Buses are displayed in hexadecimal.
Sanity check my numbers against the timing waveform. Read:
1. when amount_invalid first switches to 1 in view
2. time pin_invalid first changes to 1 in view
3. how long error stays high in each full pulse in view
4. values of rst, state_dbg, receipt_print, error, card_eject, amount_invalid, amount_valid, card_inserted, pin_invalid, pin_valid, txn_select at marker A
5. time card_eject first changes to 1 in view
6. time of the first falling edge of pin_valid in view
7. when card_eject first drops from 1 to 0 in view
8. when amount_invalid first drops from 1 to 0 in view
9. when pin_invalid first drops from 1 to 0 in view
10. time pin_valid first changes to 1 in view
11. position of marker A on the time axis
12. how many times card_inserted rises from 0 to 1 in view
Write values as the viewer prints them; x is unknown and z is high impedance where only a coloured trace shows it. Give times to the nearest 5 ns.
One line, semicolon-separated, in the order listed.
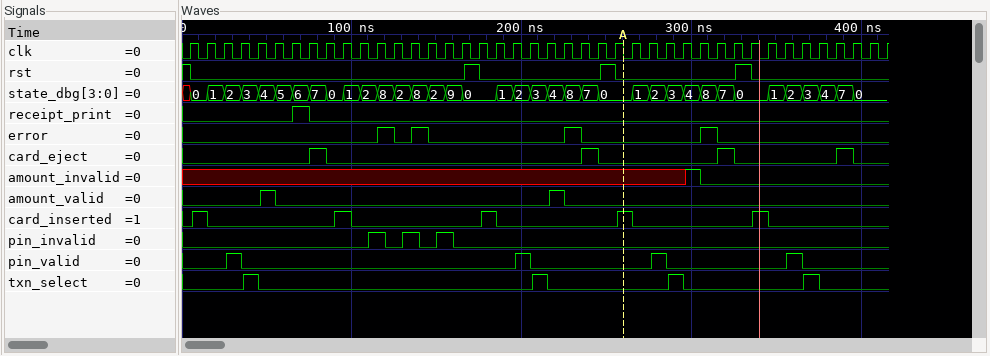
295 ns; 110 ns; 10 ns, 10 ns, 10 ns, 10 ns; rst=0, state_dbg=0, receipt_print=0, error=0, card_eject=0, amount_invalid=x, amount_valid=0, card_inserted=1, pin_invalid=0, pin_valid=0, txn_select=0; 75 ns; 35 ns; 85 ns; 305 ns; 120 ns; 25 ns; 260 ns; 5
